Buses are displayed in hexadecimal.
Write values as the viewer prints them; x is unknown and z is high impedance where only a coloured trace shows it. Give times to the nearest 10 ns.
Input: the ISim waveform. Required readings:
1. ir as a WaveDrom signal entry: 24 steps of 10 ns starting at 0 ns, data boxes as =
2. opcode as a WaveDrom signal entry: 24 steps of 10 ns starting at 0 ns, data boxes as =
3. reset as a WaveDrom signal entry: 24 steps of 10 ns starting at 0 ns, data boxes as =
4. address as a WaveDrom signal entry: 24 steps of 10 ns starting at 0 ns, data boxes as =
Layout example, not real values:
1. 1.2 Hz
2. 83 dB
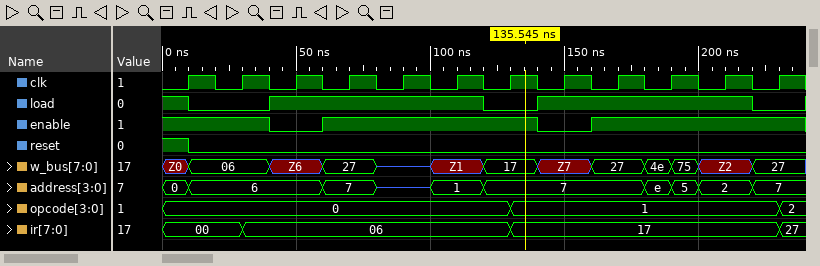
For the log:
1. {name: 'ir', wave: '=..=.........=.........=', data: '00 06 17 27'}
2. {name: 'opcode', wave: '=............=.........=', data: '0 1 2'}
3. {name: 'reset', wave: '10......................'}
4. {name: 'address', wave: '==....=.z.=.=.....===.=.', data: '0 6 7 1 7 e 5 2 7'}
